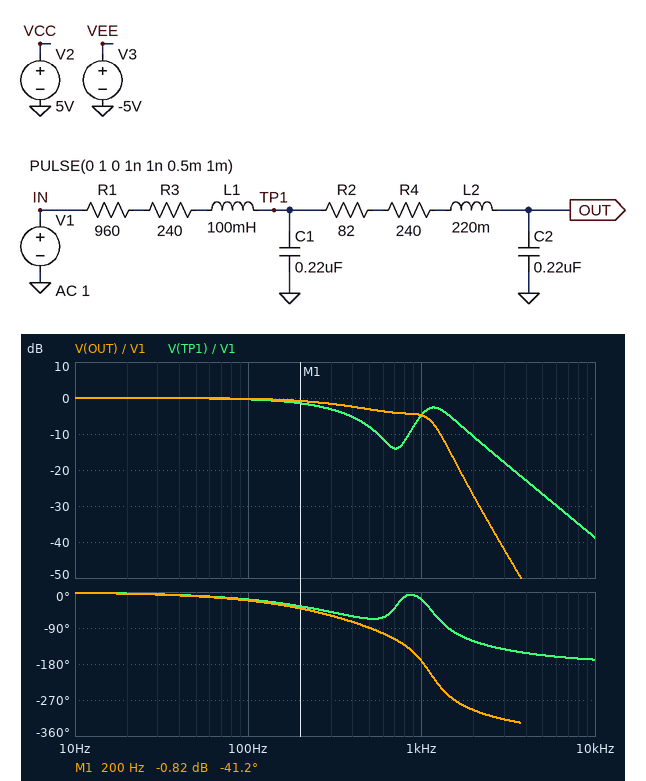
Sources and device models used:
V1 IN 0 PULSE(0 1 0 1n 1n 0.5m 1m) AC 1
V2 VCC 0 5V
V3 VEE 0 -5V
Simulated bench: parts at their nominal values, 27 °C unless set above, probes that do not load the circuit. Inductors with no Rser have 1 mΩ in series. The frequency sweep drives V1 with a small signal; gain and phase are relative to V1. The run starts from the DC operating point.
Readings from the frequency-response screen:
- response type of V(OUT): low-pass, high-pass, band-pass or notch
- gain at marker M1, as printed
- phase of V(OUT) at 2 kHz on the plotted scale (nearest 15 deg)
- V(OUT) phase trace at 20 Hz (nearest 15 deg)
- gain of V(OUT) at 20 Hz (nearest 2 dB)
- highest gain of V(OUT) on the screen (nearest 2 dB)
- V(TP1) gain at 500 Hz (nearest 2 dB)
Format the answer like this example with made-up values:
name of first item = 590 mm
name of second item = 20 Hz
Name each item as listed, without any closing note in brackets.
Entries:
response type of V(OUT): low-pass, high-pass, band-pass or notch = low-pass
gain at marker M1, as printed = -0.82 dB
phase of V(OUT) at 2 kHz on the plotted scale = -300 deg
V(OUT) phase trace at 20 Hz = 0 deg
gain of V(OUT) at 20 Hz = 0 dB
highest gain of V(OUT) on the screen = 0 dB
V(TP1) gain at 500 Hz = -8 dB
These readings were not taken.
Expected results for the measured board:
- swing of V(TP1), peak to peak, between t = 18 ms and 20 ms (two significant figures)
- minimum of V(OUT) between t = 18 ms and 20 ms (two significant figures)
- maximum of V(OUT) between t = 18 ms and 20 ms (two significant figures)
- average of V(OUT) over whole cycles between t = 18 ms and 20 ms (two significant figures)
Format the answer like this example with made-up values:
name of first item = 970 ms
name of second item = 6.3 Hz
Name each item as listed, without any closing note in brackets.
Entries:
swing of V(TP1), peak to peak, between t = 18 ms and 20 ms = 750 mV
minimum of V(OUT) between t = 18 ms and 20 ms = 130 mV
maximum of V(OUT) between t = 18 ms and 20 ms = 870 mV
average of V(OUT) over whole cycles between t = 18 ms and 20 ms = 500 mV
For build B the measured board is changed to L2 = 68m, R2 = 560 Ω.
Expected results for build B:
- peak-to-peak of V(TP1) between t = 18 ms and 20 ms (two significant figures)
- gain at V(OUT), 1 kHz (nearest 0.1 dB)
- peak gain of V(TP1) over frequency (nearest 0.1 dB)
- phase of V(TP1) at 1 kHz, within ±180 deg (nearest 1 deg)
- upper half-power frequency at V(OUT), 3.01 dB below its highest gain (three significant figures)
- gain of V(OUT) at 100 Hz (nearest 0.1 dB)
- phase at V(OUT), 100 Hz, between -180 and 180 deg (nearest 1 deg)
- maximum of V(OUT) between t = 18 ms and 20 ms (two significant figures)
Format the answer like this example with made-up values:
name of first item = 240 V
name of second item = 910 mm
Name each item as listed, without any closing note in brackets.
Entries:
peak-to-peak of V(TP1) between t = 18 ms and 20 ms = 430 mV
gain at V(OUT), 1 kHz = -11.2 dB
peak gain of V(TP1) over frequency = 0 dB
phase of V(TP1) at 1 kHz, within ±180 deg = -67 deg
upper half-power frequency at V(OUT), 3.01 dB below its highest gain = 297 Hz
gain of V(OUT) at 100 Hz = -0.5 dB
phase at V(OUT), 100 Hz, between -180 and 180 deg = -25 deg
maximum of V(OUT) between t = 18 ms and 20 ms = 680 mV
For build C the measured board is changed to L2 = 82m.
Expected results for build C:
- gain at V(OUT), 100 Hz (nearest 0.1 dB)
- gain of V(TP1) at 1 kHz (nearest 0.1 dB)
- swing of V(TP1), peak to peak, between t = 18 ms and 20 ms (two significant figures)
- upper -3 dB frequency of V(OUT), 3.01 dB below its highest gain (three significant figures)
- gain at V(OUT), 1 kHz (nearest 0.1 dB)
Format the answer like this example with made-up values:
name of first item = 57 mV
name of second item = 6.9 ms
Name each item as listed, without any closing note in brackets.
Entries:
gain at V(OUT), 100 Hz = -0.3 dB
gain of V(TP1) at 1 kHz = -14.1 dB
swing of V(TP1), peak to peak, between t = 18 ms and 20 ms = 290 mV
upper -3 dB frequency of V(OUT), 3.01 dB below its highest gain = 360 Hz
gain at V(OUT), 1 kHz = -8.6 dB
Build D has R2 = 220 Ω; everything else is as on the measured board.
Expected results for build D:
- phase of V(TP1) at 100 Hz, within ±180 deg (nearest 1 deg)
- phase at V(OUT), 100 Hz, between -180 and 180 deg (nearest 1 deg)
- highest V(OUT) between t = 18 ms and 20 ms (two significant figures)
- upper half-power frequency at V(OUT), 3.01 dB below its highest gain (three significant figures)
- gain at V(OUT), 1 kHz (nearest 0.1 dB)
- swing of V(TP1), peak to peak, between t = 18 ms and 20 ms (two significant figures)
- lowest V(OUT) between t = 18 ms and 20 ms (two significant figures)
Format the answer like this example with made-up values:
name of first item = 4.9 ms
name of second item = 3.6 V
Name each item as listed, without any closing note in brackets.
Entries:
phase of V(TP1) at 100 Hz, within ±180 deg = -19 deg
phase at V(OUT), 100 Hz, between -180 and 180 deg = -22 deg
highest V(OUT) between t = 18 ms and 20 ms = 810 mV
upper half-power frequency at V(OUT), 3.01 dB below its highest gain = 428 Hz
gain at V(OUT), 1 kHz = -6.3 dB
swing of V(TP1), peak to peak, between t = 18 ms and 20 ms = 680 mV
lowest V(OUT) between t = 18 ms and 20 ms = 190 mV
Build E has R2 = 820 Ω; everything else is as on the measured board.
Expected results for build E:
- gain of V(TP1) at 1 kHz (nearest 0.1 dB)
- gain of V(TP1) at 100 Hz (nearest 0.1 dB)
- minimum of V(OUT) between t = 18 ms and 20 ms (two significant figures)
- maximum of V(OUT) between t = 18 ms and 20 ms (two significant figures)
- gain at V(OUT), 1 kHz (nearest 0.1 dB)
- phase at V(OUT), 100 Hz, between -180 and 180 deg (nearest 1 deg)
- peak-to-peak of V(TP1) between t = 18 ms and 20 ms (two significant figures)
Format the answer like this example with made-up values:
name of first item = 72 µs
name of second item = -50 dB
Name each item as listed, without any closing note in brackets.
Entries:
gain of V(TP1) at 1 kHz = -6.0 dB
gain of V(TP1) at 100 Hz = -0.5 dB
minimum of V(OUT) between t = 18 ms and 20 ms = 310 mV
maximum of V(OUT) between t = 18 ms and 20 ms = 690 mV
gain at V(OUT), 1 kHz = -10.7 dB
phase at V(OUT), 100 Hz, between -180 and 180 deg = -27 deg
peak-to-peak of V(TP1) between t = 18 ms and 20 ms = 590 mV
